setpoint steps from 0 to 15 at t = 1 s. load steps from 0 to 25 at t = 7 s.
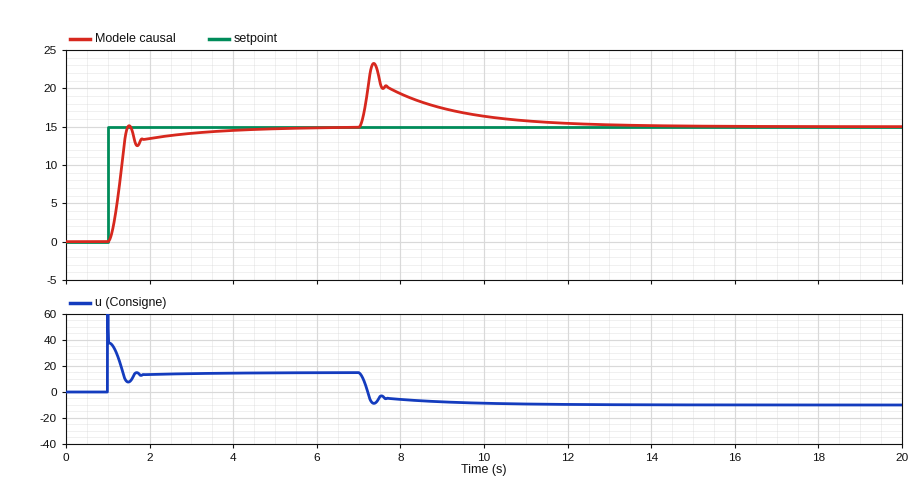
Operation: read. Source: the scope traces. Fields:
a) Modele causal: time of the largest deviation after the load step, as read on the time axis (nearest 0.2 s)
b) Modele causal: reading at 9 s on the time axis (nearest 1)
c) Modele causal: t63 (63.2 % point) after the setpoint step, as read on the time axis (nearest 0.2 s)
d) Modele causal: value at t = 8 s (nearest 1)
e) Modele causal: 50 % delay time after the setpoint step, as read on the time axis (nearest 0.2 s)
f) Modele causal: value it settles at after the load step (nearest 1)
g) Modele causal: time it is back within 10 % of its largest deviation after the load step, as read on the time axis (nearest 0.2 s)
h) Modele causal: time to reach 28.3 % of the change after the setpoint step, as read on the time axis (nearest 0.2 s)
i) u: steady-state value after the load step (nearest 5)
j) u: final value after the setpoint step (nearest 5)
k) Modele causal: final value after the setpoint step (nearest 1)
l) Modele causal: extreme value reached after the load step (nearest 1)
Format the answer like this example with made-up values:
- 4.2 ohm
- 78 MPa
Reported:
- 7.4 s
- 17
- 1.4 s
- 19
- 1.2 s
- 15
- 10.8 s
- 1.2 s
- -10
- 15
- 15
- 23
